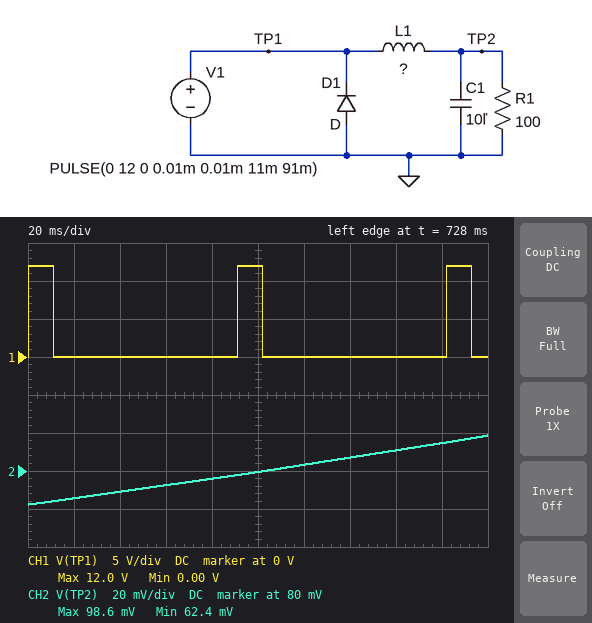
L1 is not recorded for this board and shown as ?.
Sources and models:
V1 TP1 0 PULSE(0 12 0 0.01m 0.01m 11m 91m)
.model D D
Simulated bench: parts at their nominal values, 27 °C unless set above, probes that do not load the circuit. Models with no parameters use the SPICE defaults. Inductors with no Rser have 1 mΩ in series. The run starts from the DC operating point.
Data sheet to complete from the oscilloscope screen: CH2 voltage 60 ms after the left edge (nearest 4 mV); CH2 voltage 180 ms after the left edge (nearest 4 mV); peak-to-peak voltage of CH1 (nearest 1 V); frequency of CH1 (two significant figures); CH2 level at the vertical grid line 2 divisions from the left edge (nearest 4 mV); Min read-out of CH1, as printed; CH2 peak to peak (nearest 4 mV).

72 mV
96 mV
12 V
11 Hz
68 mV
0.00 V
36 mV
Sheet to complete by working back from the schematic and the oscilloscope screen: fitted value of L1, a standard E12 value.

680 mH
